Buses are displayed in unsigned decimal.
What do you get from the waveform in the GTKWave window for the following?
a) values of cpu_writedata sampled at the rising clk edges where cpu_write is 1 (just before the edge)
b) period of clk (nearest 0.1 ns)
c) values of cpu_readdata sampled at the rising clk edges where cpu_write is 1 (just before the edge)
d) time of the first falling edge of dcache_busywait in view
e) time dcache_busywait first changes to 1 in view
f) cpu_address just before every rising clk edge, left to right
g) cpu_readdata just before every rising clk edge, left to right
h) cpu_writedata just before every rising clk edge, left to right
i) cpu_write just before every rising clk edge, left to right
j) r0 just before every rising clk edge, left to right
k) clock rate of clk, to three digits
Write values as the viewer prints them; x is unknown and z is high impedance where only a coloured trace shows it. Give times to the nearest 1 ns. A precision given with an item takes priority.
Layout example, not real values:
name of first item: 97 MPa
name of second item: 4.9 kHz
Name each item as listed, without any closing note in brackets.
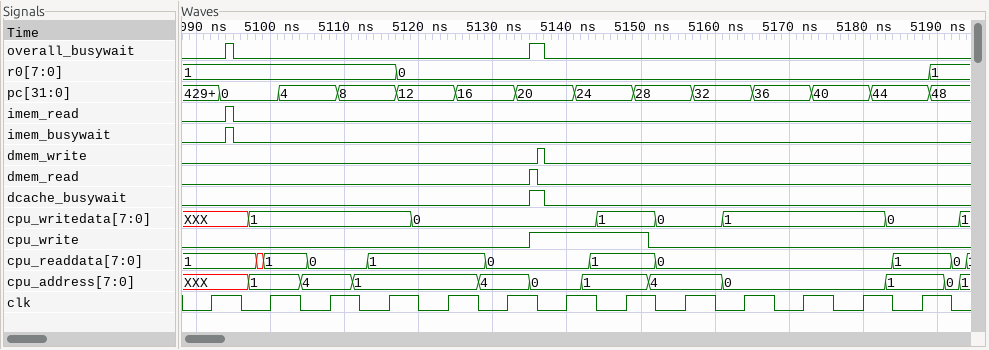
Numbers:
values of cpu_writedata sampled at the rising clk edges where cpu_write is 1: 0, 1
period of clk: 8 ns
values of cpu_readdata sampled at the rising clk edges where cpu_write is 1: 0, 1
time of the first falling edge of dcache_busywait in view: 5137 ns
time dcache_busywait first changes to 1 in view: 5135 ns
cpu_address just before every rising clk edge, left to right: XXX, 1, 4, 1, 1, 4, 0, 1, 4, 0, 0, 0, 1
cpu_readdata just before every rising clk edge, left to right: 1, 1, 0, 1, 1, 0, 0, 1, 0, 0, 0, 0, 1
cpu_writedata just before every rising clk edge, left to right: XXX, 1, 1, 1, 0, 0, 0, 1, 0, 1, 1, 1, 0
cpu_write just before every rising clk edge, left to right: 0 0 0 0 0 0 1 1 0 0 0 0 0
r0 just before every rising clk edge, left to right: 1, 1, 1, 1, 0, 0, 0, 0, 0, 0, 0, 0, 0
clock rate of clk, to three digits: 125 MHz
